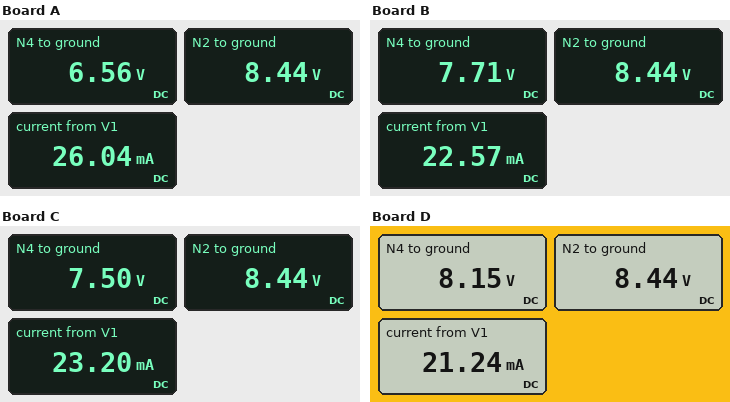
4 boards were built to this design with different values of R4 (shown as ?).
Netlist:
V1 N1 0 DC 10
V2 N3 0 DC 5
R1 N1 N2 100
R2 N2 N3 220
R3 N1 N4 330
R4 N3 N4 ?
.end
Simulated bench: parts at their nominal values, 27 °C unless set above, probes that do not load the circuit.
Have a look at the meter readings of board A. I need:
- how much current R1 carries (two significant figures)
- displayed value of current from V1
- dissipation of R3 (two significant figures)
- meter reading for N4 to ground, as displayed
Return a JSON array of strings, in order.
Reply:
["16 mA", "26.04 mA", "36 mW", "6.56 V"]
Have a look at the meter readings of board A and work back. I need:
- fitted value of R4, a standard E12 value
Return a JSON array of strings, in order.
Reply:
["150 Ω"]
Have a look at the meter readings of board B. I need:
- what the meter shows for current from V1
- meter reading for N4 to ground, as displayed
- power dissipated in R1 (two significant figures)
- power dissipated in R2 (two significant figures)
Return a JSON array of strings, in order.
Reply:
["22.57 mA", "7.71 V", "24 mW", "54 mW"]
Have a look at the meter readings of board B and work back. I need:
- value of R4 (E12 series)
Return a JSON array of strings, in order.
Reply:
["390 Ω"]
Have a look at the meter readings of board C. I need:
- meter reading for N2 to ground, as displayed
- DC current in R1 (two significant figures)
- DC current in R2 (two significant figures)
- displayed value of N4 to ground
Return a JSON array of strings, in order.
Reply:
["8.44 V", "16 mA", "16 mA", "7.50 V"]
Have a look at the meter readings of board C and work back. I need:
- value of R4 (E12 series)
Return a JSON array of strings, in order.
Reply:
["330 Ω"]
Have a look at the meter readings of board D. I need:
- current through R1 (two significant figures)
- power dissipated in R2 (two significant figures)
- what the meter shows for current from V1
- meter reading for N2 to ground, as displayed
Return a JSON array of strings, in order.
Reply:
["16 mA", "54 mW", "21.24 mA", "8.44 V"]
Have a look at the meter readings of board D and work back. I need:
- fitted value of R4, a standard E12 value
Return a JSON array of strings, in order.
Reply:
["560 Ω"]
